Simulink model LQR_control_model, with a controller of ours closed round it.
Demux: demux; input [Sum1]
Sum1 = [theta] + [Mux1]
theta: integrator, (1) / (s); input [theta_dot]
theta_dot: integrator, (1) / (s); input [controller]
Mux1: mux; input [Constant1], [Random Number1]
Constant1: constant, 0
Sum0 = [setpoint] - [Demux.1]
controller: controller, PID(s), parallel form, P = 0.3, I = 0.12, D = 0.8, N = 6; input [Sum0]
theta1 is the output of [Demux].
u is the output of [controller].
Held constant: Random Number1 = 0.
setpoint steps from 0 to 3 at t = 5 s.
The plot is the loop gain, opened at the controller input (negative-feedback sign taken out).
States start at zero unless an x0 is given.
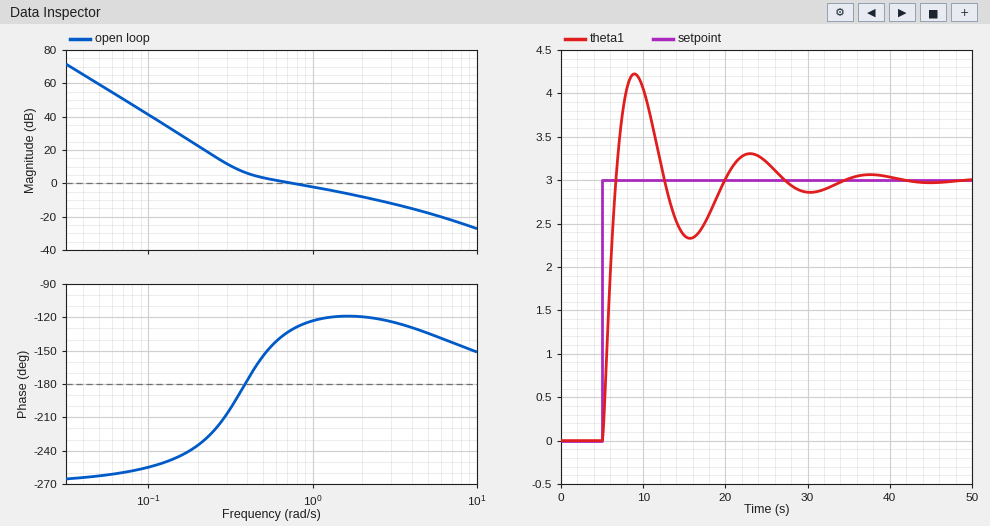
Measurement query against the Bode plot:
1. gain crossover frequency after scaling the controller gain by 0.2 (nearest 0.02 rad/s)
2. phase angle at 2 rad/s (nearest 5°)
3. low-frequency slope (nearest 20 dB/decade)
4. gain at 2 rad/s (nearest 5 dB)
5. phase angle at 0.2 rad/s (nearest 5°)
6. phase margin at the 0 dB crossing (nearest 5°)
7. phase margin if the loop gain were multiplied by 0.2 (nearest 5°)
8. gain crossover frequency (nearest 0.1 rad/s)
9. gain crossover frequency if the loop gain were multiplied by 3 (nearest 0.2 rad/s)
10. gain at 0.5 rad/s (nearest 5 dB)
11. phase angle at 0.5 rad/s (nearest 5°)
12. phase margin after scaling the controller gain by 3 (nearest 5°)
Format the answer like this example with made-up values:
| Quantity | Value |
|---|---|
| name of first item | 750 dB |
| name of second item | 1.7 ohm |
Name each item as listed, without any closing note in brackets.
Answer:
| Quantity | Value |
|---|---|
| gain crossover frequency after scaling the controller gain by 0.2 | 0.28 rad/s |
| phase angle at 2 rad/s | -120° |
| low-frequency slope | -60 dB/decade |
| gain at 2 rad/s | -10 dB |
| phase angle at 0.2 rad/s | -235° |
| phase margin at the 0 dB crossing | 50° |
| phase margin if the loop gain were multiplied by 0.2 | -35° |
| gain crossover frequency | 0.8 rad/s |
| gain crossover frequency if the loop gain were multiplied by 3 | 2.4 rad/s |
| gain at 0.5 rad/s | 5 dB |
| phase angle at 0.5 rad/s | -155° |
| phase margin after scaling the controller gain by 3 | 60° |
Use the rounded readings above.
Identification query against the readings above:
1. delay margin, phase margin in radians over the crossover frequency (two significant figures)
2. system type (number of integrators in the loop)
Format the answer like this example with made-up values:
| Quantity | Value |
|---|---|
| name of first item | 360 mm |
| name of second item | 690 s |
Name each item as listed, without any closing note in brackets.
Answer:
| Quantity | Value |
|---|---|
| delay margin, phase margin in radians over the crossover frequency | 1.1 s |
| system type | 3 |
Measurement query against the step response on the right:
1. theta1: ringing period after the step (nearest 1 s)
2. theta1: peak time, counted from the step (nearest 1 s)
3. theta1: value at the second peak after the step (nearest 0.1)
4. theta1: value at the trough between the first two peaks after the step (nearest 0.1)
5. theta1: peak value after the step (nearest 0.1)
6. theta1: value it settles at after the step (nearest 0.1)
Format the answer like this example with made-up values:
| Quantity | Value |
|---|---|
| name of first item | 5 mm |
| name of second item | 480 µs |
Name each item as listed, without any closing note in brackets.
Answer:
| Quantity | Value |
|---|---|
| theta1: ringing period after the step | 14 s |
| theta1: peak time, counted from the step | 4 s |
| theta1: value at the second peak after the step | 3.3 |
| theta1: value at the trough between the first two peaks after the step | 2.3 |
| theta1: peak value after the step | 4.2 |
| theta1: value it settles at after the step | 3.0 |
